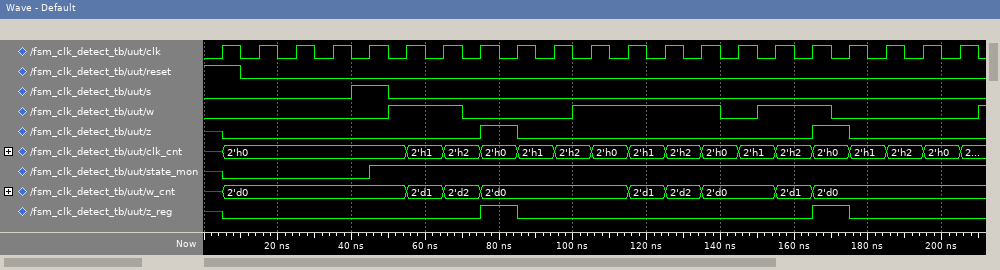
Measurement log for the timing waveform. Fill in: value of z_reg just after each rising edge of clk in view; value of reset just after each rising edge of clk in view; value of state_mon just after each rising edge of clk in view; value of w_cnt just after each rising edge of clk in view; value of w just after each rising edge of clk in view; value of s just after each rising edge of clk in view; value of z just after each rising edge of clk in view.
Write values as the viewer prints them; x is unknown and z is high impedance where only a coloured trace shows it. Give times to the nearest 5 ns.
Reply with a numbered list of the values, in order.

1. 0 0 0 0 0 0 0 1 0 0 0 0 0 0 0 0 1 0 0 0 0
2. 1 0 0 0 0 0 0 0 0 0 0 0 0 0 0 0 0 0 0 0 0
3. 0 0 0 0 1 1 1 1 1 1 1 1 1 1 1 1 1 1 1 1 1
4. 2'd0, 2'd0, 2'd0, 2'd0, 2'd0, 2'd1, 2'd2, 2'd0, 2'd0, 2'd0, 2'd0, 2'd1, 2'd2, 2'd0, 2'd0, 2'd1, 2'd0, 2'd0, 2'd0, 2'd0, 2'd0
5. 0 0 0 0 0 1 1 0 0 0 1 1 1 1 0 1 1 0 0 0 0
6. 0 0 0 0 1 0 0 0 0 0 0 0 0 0 0 0 0 0 0 0 0
7. 0 0 0 0 0 0 0 1 0 0 0 0 0 0 0 0 1 0 0 0 0
